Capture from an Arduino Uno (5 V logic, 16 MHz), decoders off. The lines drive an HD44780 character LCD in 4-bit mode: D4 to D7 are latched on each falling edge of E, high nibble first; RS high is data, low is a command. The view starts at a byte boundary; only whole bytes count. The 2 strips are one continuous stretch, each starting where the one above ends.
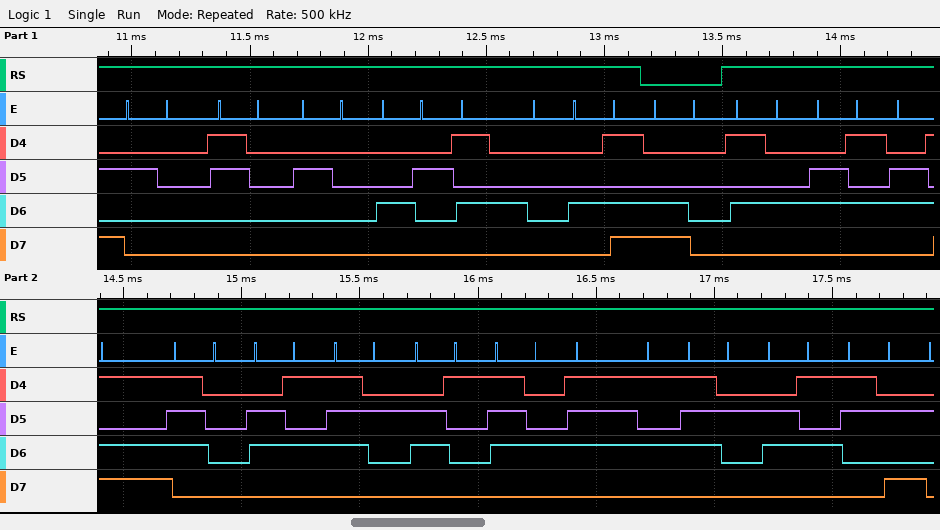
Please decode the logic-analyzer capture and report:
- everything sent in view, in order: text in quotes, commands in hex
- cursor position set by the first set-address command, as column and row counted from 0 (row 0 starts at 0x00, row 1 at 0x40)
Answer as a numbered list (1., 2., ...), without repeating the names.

1. " 0 BPM" 0xC0 "Temperature:"
2. column 0, row 1
